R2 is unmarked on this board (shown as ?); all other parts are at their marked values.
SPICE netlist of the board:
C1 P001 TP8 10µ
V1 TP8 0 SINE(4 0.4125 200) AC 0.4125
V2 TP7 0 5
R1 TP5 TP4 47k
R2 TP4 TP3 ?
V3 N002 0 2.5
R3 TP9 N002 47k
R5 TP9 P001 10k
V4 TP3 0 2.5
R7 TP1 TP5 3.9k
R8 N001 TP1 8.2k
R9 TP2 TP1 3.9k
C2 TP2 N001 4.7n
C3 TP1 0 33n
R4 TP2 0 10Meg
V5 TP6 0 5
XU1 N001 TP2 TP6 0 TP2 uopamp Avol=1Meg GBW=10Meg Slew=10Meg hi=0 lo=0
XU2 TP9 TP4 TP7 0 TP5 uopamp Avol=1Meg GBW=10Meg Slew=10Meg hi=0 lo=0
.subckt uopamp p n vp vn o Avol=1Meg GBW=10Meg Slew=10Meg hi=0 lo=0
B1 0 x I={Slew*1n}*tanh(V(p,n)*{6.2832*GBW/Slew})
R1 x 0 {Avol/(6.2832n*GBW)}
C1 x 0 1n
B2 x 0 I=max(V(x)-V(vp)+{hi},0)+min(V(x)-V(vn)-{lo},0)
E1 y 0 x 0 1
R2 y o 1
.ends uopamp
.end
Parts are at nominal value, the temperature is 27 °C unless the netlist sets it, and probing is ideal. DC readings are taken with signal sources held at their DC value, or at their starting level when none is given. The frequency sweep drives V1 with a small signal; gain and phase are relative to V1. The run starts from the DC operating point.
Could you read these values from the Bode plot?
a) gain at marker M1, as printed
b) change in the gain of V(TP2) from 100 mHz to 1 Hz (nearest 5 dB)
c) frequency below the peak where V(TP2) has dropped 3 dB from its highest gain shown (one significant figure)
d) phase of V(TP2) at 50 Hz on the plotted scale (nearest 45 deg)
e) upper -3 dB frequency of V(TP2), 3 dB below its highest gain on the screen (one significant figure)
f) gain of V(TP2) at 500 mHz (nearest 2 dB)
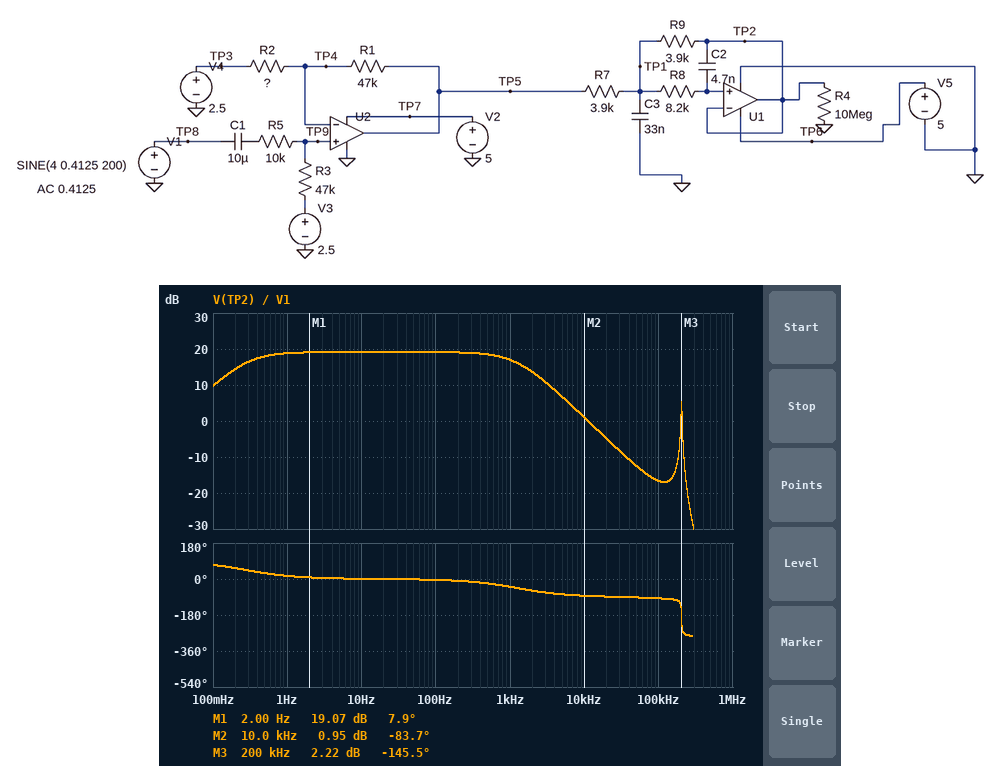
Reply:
19.07 dB
10 dB
300 mHz
0 deg
1 kHz
18 dB
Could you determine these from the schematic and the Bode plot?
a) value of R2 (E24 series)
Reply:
4.7 kΩ
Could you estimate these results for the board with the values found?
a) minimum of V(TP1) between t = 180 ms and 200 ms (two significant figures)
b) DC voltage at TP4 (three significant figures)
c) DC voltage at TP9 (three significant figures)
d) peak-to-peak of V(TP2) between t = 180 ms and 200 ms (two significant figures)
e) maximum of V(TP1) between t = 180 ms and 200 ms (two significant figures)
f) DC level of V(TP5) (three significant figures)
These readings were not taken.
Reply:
-2.9 mV
2.50 V
2.50 V
5.0 V
5.0 V
2.50 V
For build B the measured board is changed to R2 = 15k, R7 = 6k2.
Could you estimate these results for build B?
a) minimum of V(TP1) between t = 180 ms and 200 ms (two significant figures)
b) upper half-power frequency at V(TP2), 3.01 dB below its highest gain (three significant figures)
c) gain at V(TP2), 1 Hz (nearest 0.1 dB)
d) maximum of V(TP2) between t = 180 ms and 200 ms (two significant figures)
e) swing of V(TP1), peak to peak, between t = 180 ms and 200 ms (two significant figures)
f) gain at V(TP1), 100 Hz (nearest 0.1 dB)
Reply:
1.1 V
778 Hz
10.3 dB
3.9 V
2.7 V
10.6 dB
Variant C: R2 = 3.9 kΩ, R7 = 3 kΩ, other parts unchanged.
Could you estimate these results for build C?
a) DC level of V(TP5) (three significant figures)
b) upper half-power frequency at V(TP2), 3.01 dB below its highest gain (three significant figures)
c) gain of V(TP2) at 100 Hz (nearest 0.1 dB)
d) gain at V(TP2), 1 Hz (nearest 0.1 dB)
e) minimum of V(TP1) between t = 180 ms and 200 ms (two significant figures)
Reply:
2.50 V
1.61 kHz
20.6 dB
20.3 dB
-4.2 mV
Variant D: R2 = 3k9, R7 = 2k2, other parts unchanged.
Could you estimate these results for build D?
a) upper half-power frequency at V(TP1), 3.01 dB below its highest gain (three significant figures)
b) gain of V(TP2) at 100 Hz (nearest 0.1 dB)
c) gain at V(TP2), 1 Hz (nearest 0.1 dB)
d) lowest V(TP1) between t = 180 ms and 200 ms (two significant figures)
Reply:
2.19 kHz
20.6 dB
20.3 dB
-4.7 mV
